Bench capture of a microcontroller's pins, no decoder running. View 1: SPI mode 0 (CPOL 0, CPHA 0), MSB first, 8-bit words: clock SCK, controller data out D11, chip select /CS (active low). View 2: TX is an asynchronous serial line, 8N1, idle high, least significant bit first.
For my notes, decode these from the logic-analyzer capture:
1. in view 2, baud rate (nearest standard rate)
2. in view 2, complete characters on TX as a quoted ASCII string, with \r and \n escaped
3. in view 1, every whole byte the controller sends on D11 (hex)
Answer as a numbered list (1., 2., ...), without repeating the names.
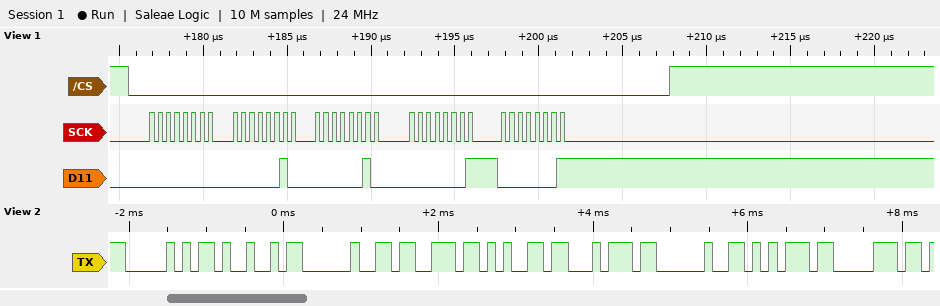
1. 9600 baud
2. "PI set up"
3. 00 02 02 01 01
